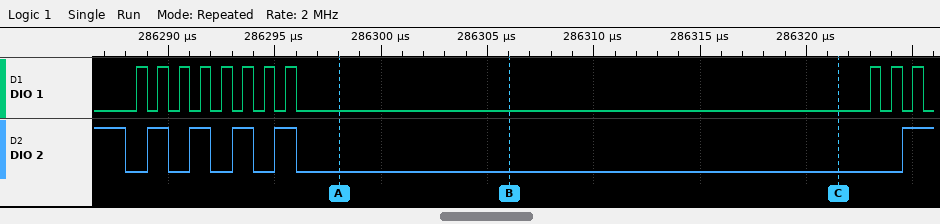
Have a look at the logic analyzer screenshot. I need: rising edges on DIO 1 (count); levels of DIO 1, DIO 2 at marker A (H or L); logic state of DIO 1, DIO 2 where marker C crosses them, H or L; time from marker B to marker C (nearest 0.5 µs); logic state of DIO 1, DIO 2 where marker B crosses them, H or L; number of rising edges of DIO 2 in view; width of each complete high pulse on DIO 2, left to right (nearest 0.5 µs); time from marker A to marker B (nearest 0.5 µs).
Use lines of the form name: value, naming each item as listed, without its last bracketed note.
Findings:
rising edges on DIO 1: 11
levels of DIO 1, DIO 2 at marker A: DIO 1=L, DIO 2=L
logic state of DIO 1, DIO 2 where marker C crosses them, H or L: DIO 1=L, DIO 2=L
time from marker B to marker C: 15.5 µs
logic state of DIO 1, DIO 2 where marker B crosses them, H or L: DIO 1=L, DIO 2=L
number of rising edges of DIO 2 in view: 5
width of each complete high pulse on DIO 2, left to right: 1 µs, 1 µs, 1 µs, 1 µs
time from marker A to marker B: 8 µs
